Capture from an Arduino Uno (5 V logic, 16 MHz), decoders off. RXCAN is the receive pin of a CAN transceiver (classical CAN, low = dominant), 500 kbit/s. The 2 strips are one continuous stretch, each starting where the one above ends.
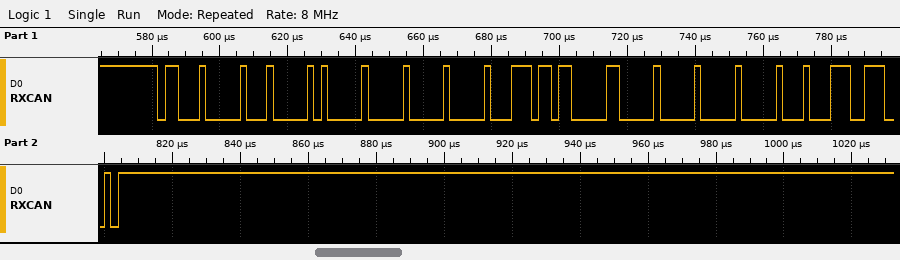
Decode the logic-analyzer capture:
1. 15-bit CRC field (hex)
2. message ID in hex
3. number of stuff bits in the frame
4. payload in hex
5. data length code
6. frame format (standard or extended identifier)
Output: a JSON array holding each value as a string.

["0x239C", "0x620", "11", "10 00 00 1D B0 40 00 00", "8", "standard"]
